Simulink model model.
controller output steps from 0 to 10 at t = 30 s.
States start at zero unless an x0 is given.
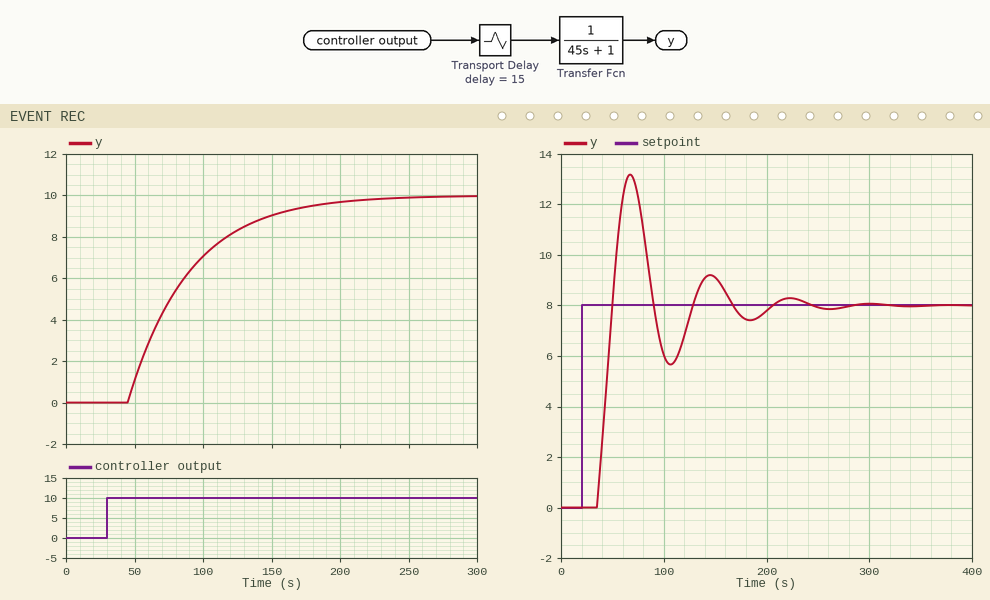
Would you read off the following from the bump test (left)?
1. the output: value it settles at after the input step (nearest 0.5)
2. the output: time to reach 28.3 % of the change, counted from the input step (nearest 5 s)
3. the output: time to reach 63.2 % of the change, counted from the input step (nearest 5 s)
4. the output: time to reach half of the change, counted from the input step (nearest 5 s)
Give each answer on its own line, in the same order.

10.0
30 s
60 s
45 s
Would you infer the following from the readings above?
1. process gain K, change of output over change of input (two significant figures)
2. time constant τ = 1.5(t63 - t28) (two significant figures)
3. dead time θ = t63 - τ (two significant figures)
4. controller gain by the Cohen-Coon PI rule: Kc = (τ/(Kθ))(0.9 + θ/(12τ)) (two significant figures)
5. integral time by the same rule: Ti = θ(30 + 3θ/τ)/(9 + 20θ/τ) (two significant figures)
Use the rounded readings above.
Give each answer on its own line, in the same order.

1.0
45 s
15 s
2.8
30 s
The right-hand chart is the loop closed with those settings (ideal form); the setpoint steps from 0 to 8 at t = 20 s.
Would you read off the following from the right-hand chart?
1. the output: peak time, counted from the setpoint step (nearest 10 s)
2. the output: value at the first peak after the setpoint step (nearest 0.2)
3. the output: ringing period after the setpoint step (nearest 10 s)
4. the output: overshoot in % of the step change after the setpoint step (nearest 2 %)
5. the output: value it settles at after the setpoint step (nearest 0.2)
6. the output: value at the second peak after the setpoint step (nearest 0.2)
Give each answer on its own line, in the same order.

50 s
13.2
80 s
64 %
8.0
9.2
